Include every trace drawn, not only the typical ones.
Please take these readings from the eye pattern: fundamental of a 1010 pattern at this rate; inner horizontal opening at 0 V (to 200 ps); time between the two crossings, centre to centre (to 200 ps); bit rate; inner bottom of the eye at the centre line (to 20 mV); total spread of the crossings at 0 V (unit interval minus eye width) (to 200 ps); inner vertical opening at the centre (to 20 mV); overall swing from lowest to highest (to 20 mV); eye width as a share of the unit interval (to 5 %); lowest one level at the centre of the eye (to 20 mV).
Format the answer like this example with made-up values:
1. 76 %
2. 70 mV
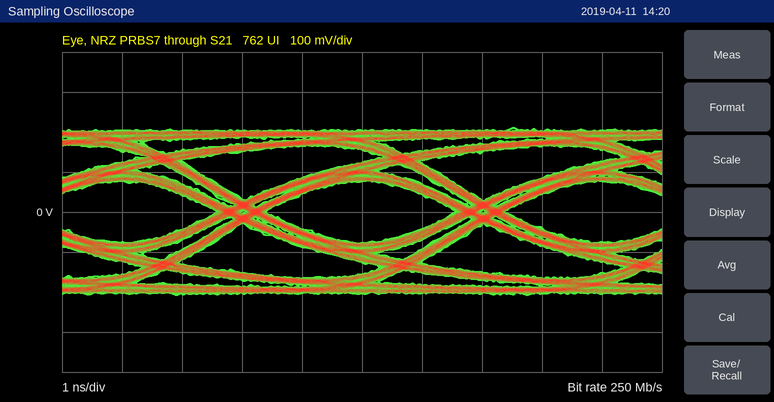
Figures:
1. 125 MHz
2. 3.2 ns
3. 4.0 ns
4. 250 Mb/s
5. -80 mV
6. 800 ps
7. 160 mV
8. 420 mV
9. 80 %
10. 80 mV
